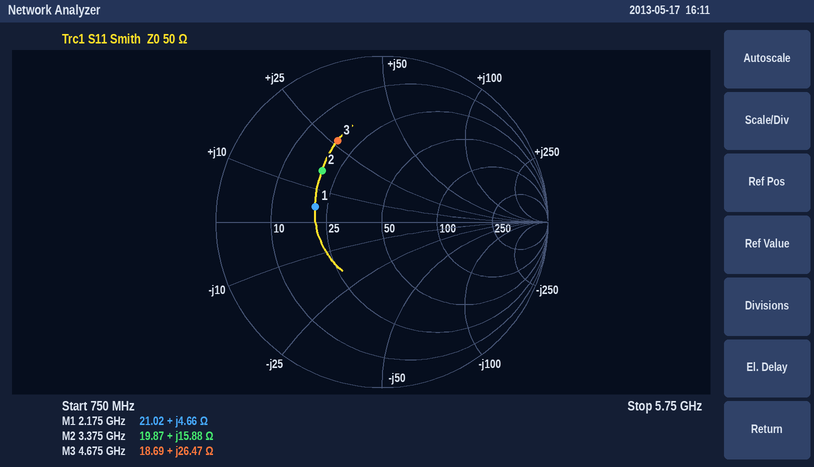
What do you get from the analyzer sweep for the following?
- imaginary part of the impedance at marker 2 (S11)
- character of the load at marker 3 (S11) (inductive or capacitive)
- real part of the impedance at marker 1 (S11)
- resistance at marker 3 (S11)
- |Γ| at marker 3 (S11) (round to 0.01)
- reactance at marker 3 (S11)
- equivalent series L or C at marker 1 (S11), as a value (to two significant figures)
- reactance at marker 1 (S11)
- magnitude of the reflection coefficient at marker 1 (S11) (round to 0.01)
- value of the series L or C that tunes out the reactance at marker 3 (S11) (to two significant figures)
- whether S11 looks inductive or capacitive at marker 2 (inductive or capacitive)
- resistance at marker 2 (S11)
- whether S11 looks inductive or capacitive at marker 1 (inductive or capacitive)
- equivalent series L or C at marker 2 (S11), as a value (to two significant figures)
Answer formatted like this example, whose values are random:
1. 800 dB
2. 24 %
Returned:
1. +15.88 Ω
2. inductive
3. 21.02 Ω
4. 18.69 Ω
5. 0.56
6. +26.47 Ω
7. 340 pH
8. +4.66 Ω
9. 0.41
10. 1.3 pF
11. inductive
12. 19.87 Ω
13. inductive
14. 750 pH
